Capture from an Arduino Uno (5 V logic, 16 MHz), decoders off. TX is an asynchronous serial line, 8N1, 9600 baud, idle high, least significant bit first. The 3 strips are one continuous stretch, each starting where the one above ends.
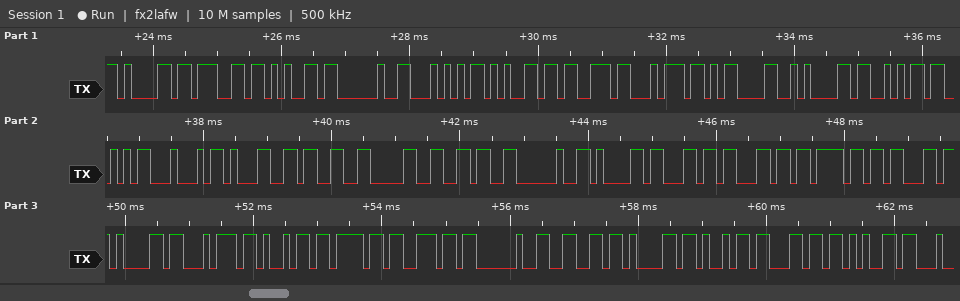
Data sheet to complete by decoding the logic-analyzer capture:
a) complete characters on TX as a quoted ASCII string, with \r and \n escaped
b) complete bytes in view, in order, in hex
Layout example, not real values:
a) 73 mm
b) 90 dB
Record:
a) "age Test\r\nSSD1306 allocation faile"
b) 0x61 0x67 0x65 0x20 0x54 0x65 0x73 0x74 0x0D 0x0A 0x53 0x53 0x44 0x31 0x33 0x30 0x36 0x20 0x61 0x6C 0x6C 0x6F 0x63 0x61 0x74 0x69 0x6F 0x6E 0x20 0x66 0x61 0x69 0x6C 0x65
